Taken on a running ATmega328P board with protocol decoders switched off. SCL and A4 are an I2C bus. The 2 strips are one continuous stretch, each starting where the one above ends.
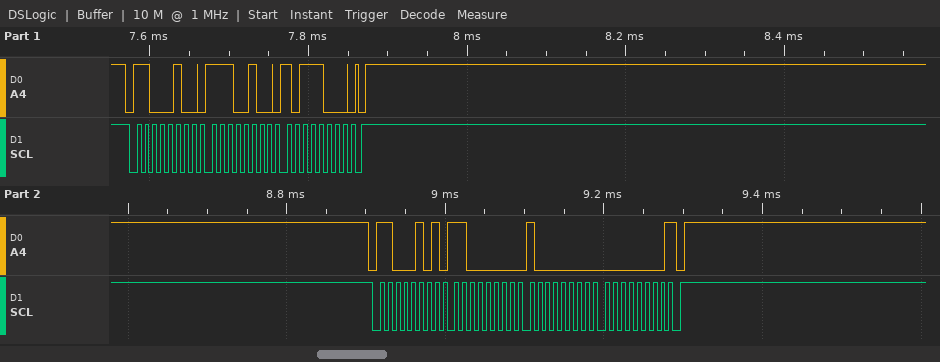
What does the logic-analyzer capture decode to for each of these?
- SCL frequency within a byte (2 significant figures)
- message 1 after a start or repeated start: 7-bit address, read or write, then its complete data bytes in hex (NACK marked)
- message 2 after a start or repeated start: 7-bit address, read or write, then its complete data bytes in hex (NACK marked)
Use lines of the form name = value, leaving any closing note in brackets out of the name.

SCL frequency within a byte = 100 kHz
message 1 after a start or repeated start: 7-bit address, read or write, then its complete data bytes in hex = 0x62 write: E4 B8
message 2 after a start or repeated start: 7-bit address, read or write, then its complete data bytes in hex = 0x62 read: C0 80 00 NACK
